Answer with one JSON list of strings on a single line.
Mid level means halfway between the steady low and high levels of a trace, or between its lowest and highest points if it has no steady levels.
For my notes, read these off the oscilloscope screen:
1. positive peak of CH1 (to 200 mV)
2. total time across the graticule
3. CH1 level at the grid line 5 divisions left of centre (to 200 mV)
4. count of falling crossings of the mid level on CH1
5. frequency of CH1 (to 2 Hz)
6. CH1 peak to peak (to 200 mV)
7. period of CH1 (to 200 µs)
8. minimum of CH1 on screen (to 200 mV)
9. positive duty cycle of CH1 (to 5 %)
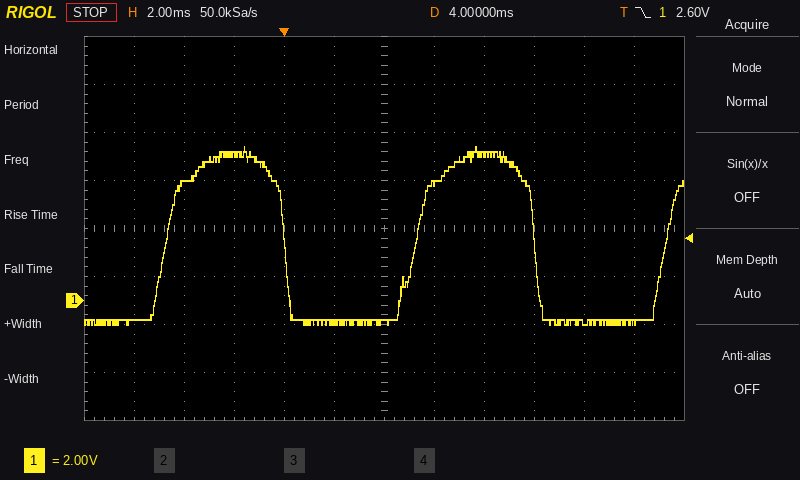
["6.4 V", "24 ms", "-800 mV", "2", "100 Hz", "7.4 V", "10.0 ms", "-1.0 V", "45 %"]
